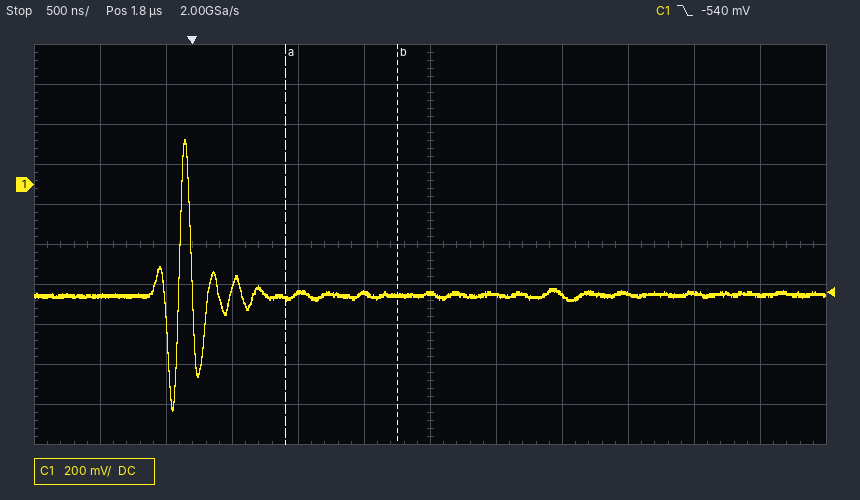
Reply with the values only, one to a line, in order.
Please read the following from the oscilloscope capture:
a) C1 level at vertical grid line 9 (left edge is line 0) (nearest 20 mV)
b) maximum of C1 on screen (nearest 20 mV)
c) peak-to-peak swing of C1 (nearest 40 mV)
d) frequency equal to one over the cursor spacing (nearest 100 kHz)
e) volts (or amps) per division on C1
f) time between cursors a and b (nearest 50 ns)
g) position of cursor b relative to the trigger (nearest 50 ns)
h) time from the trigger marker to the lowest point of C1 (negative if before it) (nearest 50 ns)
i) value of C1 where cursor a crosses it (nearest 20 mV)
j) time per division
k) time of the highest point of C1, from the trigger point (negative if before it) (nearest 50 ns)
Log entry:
-540 mV
220 mV
1.36 V
1.2 MHz
200 mV
850 ns
+1.55 µs
-150 ns
-560 mV
500 ns
-50 ns
